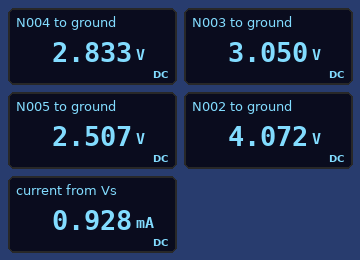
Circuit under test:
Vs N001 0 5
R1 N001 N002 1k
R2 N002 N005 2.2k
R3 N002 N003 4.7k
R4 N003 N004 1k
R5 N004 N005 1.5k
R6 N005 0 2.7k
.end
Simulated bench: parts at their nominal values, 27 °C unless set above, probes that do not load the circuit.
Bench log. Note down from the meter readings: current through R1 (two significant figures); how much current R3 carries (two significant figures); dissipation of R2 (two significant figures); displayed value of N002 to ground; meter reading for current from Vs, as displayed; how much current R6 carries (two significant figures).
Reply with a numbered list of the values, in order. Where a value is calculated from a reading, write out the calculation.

1. (5 V - 4.072 V) / 1 kΩ = 930 µA
2. (4.072 V - 3.05 V) / 4.7 kΩ = 220 µA
3. (4.072 V - 2.507 V)^2 / 2.2 kΩ = 1.1 mW
4. 4.072 V
5. 0.928 mA
6. (2.507 V) / 2.7 kΩ = 930 µA
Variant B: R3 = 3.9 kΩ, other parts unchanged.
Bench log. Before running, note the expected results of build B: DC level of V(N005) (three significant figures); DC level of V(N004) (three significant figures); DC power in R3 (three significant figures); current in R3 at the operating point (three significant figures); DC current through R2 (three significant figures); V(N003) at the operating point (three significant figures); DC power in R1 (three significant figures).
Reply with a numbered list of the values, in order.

1. 2.53 V
2. 2.89 V
3. 224 µW
4. 240 µA
5. 697 µA
6. 3.13 V
7. 878 µW
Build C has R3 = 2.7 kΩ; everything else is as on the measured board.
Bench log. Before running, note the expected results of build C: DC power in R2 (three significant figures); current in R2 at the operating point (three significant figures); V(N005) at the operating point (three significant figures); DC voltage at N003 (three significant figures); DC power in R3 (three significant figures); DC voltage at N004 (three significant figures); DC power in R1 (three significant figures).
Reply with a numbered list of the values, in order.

1. 987 µW
2. 670 µA
3. 2.57 V
4. 3.28 V
5. 217 µW
6. 3.00 V
7. 908 µW
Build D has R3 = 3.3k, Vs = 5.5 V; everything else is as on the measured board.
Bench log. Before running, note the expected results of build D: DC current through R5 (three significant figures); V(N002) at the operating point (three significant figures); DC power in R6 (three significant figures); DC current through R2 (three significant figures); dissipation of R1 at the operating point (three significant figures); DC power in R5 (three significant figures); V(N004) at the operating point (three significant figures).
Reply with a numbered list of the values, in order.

1. 286 µA
2. 4.46 V
3. 2.91 mW
4. 753 µA
5. 1.08 mW
6. 122 µW
7. 3.23 V
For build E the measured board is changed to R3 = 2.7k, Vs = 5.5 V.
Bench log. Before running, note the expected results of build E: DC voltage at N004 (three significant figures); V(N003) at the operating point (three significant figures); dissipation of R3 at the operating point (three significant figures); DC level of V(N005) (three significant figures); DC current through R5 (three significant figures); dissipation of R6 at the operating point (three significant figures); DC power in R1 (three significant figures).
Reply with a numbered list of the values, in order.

1. 3.30 V
2. 3.61 V
3. 262 µW
4. 2.83 V
5. 312 µA
6. 2.97 mW
7. 1.10 mW
